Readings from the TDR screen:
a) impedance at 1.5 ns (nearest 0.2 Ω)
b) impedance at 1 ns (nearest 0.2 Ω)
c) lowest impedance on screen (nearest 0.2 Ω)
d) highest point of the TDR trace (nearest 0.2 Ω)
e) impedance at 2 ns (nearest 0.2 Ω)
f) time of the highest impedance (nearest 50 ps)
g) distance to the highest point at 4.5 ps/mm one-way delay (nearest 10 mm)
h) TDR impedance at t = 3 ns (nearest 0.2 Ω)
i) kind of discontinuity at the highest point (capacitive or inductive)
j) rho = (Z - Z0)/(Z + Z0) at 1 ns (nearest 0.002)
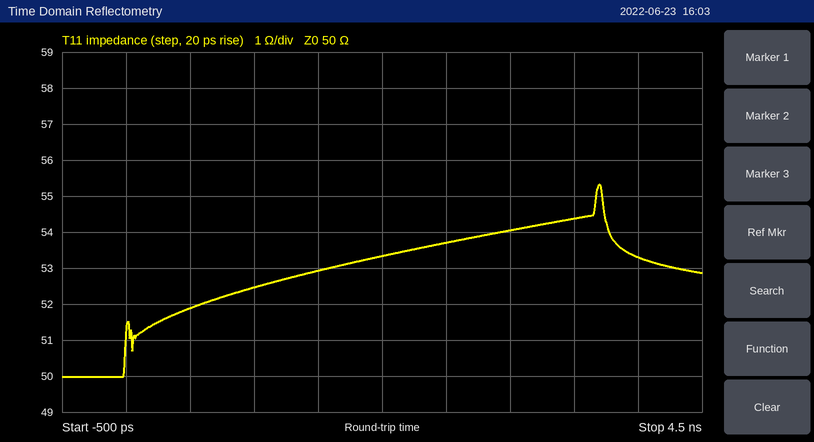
53.0 Ω
52.4 Ω
50.0 Ω
55.4 Ω
53.4 Ω
3.70 ns
410 mm
54.0 Ω
inductive
+0.024
